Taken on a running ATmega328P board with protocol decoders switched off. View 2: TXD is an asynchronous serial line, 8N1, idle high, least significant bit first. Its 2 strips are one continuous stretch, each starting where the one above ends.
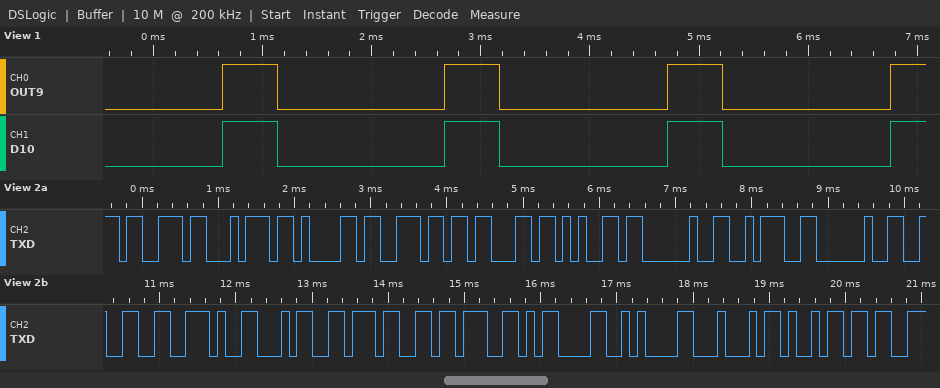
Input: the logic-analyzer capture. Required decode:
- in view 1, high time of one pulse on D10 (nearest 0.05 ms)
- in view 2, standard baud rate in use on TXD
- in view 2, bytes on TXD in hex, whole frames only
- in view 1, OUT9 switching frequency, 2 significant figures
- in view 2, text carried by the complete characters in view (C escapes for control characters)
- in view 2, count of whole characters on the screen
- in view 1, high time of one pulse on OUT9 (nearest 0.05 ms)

0.50 ms
9600 baud
73 74 61 6E 63 65 20 3A 20 32 2E 34 37 3B 0D 0A 44 69
490 Hz
"stance : 2.47;\r\nDi"
18
0.50 ms
